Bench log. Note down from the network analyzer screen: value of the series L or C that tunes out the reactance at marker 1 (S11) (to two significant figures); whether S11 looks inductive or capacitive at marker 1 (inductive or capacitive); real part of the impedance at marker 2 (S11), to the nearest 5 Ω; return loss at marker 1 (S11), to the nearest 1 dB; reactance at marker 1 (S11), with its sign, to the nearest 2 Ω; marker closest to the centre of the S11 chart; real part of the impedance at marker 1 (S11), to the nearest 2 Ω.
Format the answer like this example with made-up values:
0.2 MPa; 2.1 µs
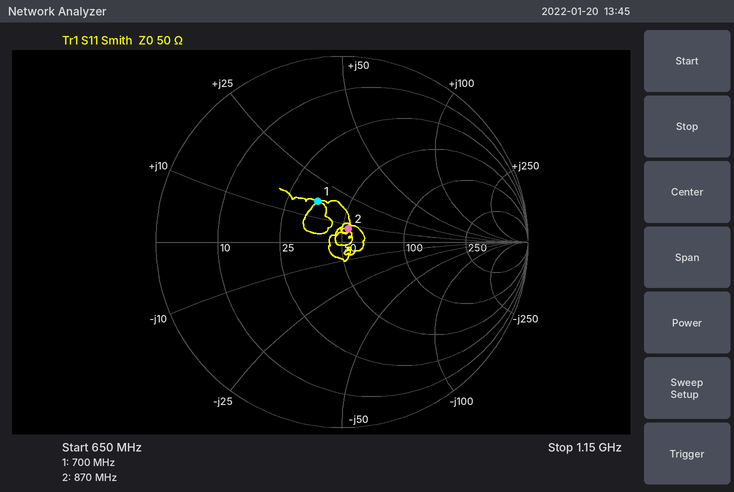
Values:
14 pF; inductive; 55 Ω; 12 dB; +16 Ω; marker 2; 36 Ω
